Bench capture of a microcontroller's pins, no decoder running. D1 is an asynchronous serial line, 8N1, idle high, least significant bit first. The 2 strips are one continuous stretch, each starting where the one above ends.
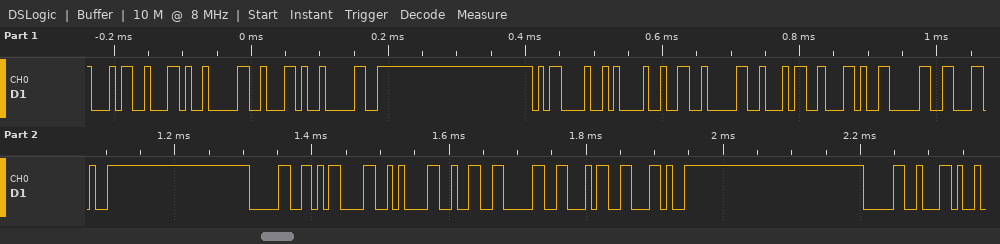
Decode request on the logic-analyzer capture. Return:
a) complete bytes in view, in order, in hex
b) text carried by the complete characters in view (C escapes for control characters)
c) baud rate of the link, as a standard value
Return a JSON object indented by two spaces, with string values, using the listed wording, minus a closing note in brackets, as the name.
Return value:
{
  "complete bytes in view, in order, in hex": "34 2C 30 2C 30 0D 0A 32 30 34 2C 30 2C 30 0D 0A 32 30 34 2C 30 2C",
  "text carried by the complete characters in view": "\"4,0,0\\r\\n204,0,0\\r\\n204,0,\"",
  "baud rate of the link, as a standard value": "115200 baud"
}
